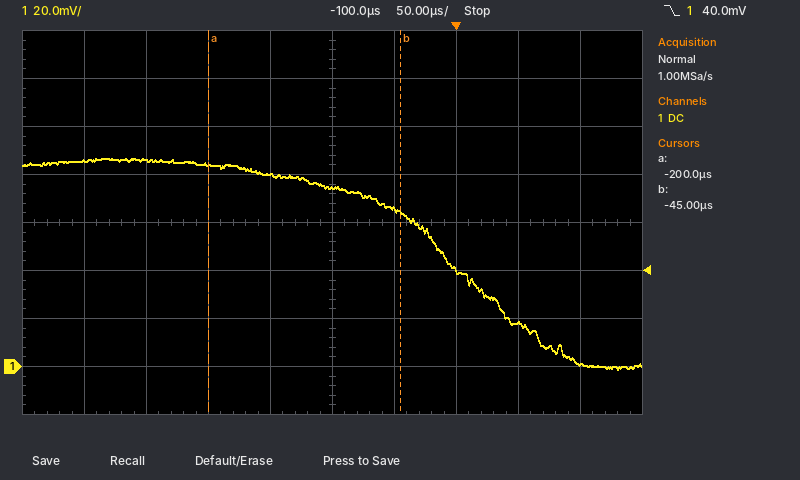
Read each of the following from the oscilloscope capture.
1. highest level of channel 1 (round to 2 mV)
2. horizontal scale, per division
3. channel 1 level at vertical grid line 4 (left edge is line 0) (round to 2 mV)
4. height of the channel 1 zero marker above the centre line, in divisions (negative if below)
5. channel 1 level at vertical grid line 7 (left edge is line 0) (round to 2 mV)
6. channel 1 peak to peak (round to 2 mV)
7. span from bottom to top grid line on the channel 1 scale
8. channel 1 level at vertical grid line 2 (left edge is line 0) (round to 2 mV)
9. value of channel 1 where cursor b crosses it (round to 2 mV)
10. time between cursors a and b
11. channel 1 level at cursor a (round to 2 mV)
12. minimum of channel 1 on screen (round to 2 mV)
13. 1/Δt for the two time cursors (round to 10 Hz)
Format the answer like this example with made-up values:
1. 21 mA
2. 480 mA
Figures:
1. 86 mV
2. 50 µs
3. 80 mV
4. -3.0 div
5. 40 mV
6. 88 mV
7. 160 mV
8. 86 mV
9. 64 mV
10. 155 µs
11. 84 mV
12. -2 mV
13. 6.45 kHz
